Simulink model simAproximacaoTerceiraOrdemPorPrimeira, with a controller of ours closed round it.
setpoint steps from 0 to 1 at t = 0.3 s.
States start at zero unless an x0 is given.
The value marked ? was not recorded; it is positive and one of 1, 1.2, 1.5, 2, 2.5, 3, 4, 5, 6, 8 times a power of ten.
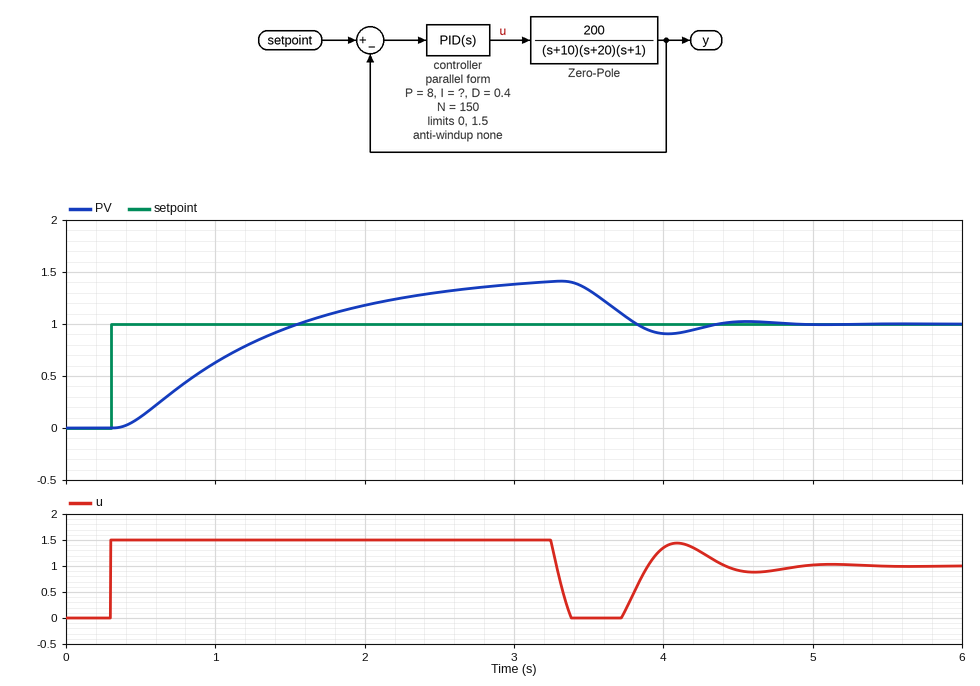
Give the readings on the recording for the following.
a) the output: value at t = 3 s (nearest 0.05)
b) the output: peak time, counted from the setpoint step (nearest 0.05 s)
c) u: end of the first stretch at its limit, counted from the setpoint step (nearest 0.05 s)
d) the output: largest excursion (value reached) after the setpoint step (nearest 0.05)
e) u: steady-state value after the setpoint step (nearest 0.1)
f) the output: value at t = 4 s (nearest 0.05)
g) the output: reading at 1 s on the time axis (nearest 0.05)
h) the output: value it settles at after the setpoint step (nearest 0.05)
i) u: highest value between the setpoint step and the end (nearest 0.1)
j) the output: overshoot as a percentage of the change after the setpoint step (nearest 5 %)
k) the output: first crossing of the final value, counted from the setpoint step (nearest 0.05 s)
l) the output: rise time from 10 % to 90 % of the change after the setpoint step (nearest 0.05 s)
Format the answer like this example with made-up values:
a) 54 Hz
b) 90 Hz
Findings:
a) 1.40
b) 3.00 s
c) 2.95 s
d) 1.40
e) 1.0
f) 0.90
g) 0.65
h) 1.00
i) 1.5
j) 40 %
k) 1.25 s
l) 0.90 s
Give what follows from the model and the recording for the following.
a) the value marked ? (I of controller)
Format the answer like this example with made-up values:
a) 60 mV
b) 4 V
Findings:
a) 30
